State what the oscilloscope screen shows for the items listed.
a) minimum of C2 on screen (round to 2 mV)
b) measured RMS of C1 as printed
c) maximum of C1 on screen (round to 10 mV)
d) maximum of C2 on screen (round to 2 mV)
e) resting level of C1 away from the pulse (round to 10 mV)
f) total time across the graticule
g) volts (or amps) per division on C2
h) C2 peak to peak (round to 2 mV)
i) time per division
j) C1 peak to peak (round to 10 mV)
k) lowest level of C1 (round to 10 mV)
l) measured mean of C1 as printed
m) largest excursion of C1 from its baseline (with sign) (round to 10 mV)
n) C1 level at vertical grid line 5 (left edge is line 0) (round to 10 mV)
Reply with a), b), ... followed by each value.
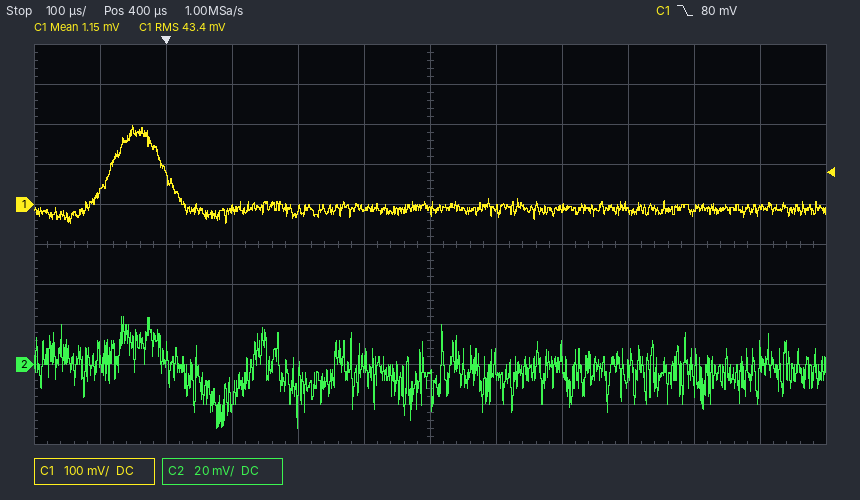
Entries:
a) -32 mV
b) 43.4 mV
c) 200 mV
d) 24 mV
e) -10 mV
f) 1.2 ms
g) 20 mV
h) 56 mV
i) 100 µs
j) 250 mV
k) -50 mV
l) 1.15 mV
m) +210 mV
n) -10 mV
